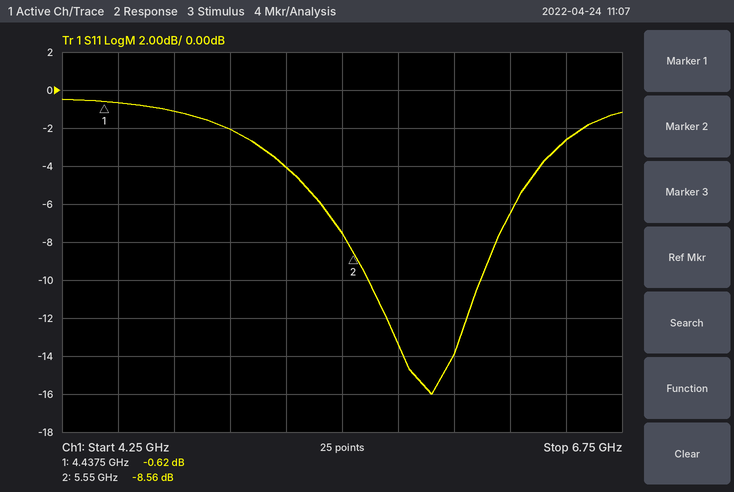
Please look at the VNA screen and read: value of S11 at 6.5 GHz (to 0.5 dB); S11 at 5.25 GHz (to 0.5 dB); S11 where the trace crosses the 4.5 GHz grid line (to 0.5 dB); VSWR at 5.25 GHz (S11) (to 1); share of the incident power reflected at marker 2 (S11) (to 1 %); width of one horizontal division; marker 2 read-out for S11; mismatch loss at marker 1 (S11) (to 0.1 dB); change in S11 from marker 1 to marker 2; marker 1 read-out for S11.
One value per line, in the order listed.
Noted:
-2.5 dB
-4.0 dB
-0.5 dB
4
14 %
250 MHz
-8.56 dB
8.8 dB
-7.94 dB
-0.62 dB
